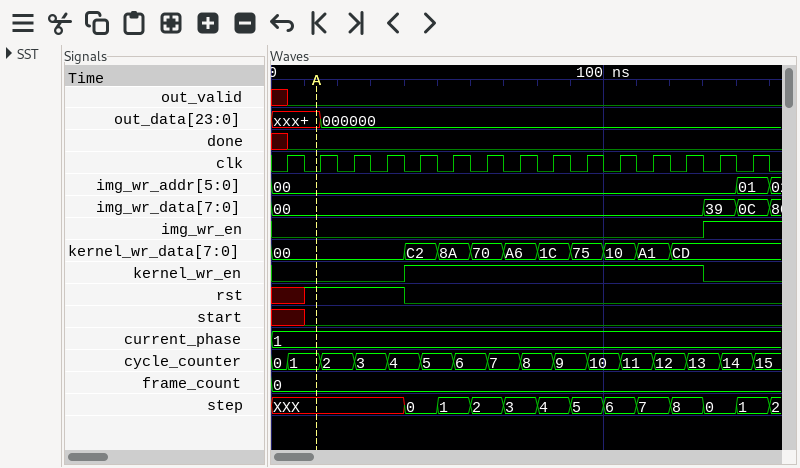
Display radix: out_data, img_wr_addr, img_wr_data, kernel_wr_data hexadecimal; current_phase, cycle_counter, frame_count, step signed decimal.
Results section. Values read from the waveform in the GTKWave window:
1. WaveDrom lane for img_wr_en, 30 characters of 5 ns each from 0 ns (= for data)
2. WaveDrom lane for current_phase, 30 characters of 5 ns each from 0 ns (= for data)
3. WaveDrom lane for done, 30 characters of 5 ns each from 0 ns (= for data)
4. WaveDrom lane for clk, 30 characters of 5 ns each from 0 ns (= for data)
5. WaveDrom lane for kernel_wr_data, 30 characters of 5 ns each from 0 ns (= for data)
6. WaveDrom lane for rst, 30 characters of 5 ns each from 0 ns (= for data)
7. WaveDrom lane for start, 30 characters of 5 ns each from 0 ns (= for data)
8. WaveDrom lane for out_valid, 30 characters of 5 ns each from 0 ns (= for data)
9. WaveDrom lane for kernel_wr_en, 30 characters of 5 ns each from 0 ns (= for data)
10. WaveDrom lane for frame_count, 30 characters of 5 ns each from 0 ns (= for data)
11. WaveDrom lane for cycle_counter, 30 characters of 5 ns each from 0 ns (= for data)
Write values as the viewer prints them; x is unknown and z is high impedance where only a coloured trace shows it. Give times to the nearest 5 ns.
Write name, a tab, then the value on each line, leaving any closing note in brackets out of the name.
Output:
WaveDrom lane for img_wr_en, 30 characters of 5 ns each from 0 ns	{name: 'img_wr_en', wave: '0.........................1...'}
WaveDrom lane for current_phase, 30 characters of 5 ns each from 0 ns	{name: 'current_phase', wave: '=.............................', data: '1'}
WaveDrom lane for done, 30 characters of 5 ns each from 0 ns	{name: 'done', wave: 'x0............................'}
WaveDrom lane for clk, 30 characters of 5 ns each from 0 ns	{name: 'clk', wave: '010101010101010101010101010101'}
WaveDrom lane for kernel_wr_data, 30 characters of 5 ns each from 0 ns	{name: 'kernel_wr_data', wave: '=.......=.=.=.=.=.=.=.=.=.....', data: '00 C2 8A 70 A6 1C 75 10 A1 CD'}
WaveDrom lane for rst, 30 characters of 5 ns each from 0 ns	{name: 'rst', wave: 'x.1.....0.....................'}
WaveDrom lane for start, 30 characters of 5 ns each from 0 ns	{name: 'start', wave: 'x.0...........................'}
WaveDrom lane for out_valid, 30 characters of 5 ns each from 0 ns	{name: 'out_valid', wave: 'x0............................'}
WaveDrom lane for kernel_wr_en, 30 characters of 5 ns each from 0 ns	{name: 'kernel_wr_en', wave: '0.......1.................0...'}
WaveDrom lane for frame_count, 30 characters of 5 ns each from 0 ns	{name: 'frame_count', wave: '=.............................', data: '0'}
WaveDrom lane for cycle_counter, 30 characters of 5 ns each from 0 ns	{name: 'cycle_counter', wave: '==.=.=.=.=.=.=.=.=.=.=.=.=.=.=', data: '0 1 2 3 4 5 6 7 8 9 10 11 12 13 14 15'}
